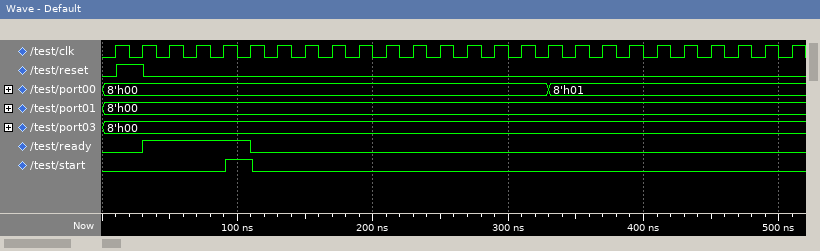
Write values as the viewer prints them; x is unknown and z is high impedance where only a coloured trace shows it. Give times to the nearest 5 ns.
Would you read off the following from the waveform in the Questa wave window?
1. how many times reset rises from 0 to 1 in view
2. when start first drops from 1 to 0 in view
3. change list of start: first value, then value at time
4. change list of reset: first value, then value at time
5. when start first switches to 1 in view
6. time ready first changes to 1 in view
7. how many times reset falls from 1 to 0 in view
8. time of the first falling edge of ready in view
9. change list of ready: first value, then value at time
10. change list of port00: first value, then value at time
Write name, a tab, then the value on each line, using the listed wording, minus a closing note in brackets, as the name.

how many times reset rises from 0 to 1 in view	1
when start first drops from 1 to 0 in view	110 ns
change list of start: first value, then value at time	0, 1 at 90 ns, 0 at 110 ns
change list of reset: first value, then value at time	0, 1 at 10 ns, 0 at 30 ns
when start first switches to 1 in view	90 ns
time ready first changes to 1 in view	30 ns
how many times reset falls from 1 to 0 in view	1
time of the first falling edge of ready in view	110 ns
change list of ready: first value, then value at time	0, 1 at 30 ns, 0 at 110 ns
change list of port00: first value, then value at time	8'h00, 8'h01 at 330 ns
